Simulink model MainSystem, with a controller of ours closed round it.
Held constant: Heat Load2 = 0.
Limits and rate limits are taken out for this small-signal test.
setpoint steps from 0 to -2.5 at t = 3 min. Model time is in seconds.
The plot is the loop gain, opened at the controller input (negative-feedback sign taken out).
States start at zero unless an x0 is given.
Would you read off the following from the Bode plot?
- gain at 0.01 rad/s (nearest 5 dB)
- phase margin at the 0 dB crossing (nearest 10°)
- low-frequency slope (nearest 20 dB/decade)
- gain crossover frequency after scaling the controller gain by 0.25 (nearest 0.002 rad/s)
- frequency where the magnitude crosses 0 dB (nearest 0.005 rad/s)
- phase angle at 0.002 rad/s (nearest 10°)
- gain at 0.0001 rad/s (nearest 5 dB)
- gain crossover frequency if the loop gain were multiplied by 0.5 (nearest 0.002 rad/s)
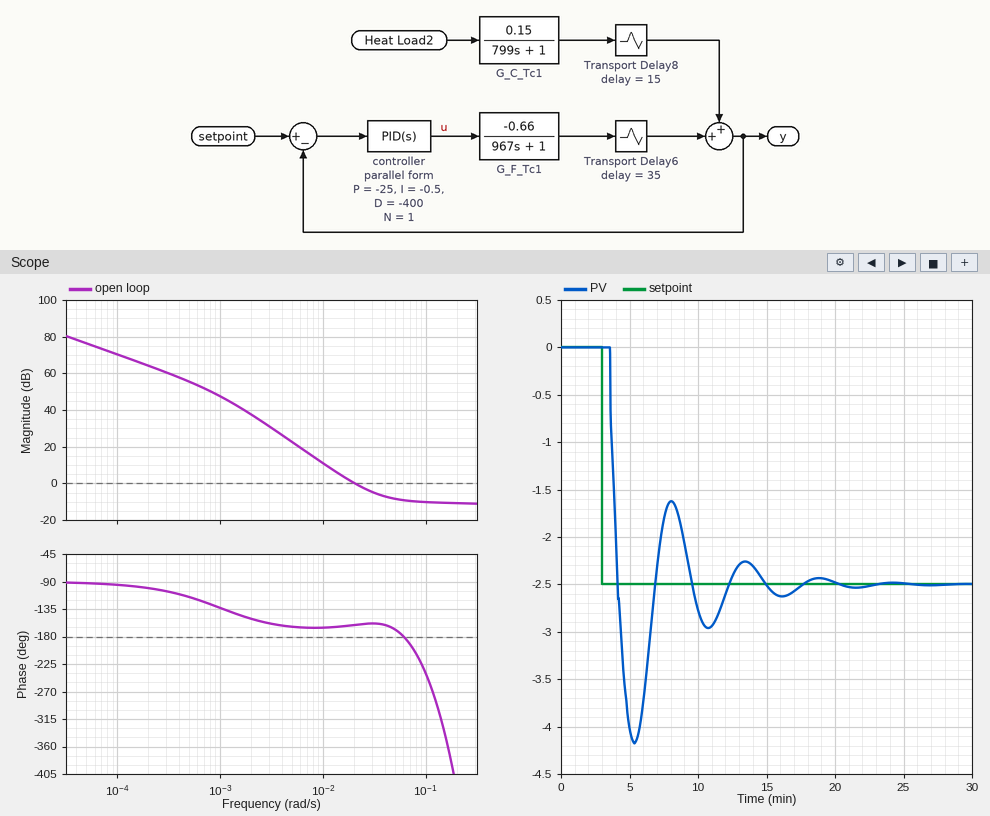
10 dB
20°
-20 dB/decade
0.010 rad/s
0.020 rad/s
-150°
70 dB
0.014 rad/s
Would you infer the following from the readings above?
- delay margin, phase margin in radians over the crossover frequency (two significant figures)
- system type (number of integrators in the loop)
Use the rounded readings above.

17 s
1
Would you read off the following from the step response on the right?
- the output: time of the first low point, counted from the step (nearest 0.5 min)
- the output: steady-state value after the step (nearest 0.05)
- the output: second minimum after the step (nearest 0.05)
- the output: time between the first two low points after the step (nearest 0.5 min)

2.5 min
-2.50
-2.95
5.5 min
